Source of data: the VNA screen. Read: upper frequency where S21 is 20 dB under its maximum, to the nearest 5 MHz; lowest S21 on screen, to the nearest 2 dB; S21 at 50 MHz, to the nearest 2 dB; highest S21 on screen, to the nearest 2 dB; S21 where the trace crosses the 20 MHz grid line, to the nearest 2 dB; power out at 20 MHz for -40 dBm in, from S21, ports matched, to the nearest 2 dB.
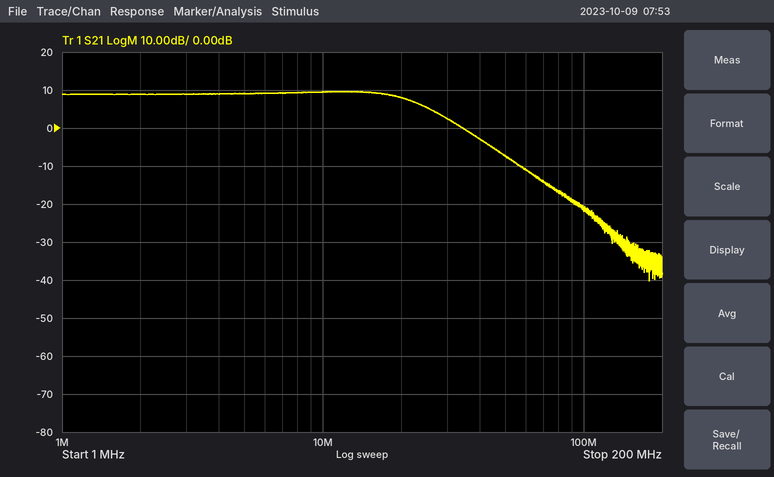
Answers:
60 MHz
-40 dB
-8 dB
10 dB
8 dB
-32 dBm
